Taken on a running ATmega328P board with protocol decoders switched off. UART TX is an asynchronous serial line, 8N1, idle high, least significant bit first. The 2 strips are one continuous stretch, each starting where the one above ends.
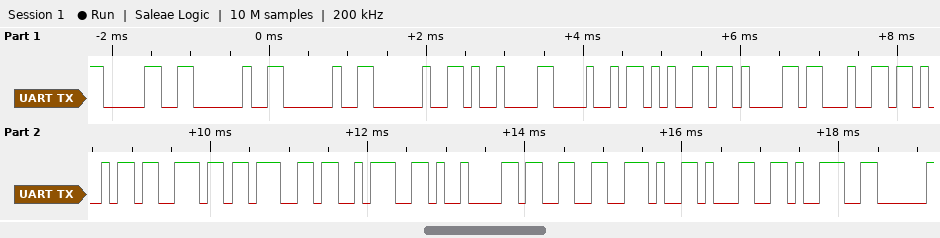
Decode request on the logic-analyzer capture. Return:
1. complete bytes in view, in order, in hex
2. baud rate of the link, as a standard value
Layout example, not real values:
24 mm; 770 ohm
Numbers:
0x30 0x20 0x20 0x20 0x09 0x48 0x65 0x61 0x64 0x69 0x6E 0x67 0x3A 0x09 0x33 0x2E 0x31 0x39; 9600 baud
